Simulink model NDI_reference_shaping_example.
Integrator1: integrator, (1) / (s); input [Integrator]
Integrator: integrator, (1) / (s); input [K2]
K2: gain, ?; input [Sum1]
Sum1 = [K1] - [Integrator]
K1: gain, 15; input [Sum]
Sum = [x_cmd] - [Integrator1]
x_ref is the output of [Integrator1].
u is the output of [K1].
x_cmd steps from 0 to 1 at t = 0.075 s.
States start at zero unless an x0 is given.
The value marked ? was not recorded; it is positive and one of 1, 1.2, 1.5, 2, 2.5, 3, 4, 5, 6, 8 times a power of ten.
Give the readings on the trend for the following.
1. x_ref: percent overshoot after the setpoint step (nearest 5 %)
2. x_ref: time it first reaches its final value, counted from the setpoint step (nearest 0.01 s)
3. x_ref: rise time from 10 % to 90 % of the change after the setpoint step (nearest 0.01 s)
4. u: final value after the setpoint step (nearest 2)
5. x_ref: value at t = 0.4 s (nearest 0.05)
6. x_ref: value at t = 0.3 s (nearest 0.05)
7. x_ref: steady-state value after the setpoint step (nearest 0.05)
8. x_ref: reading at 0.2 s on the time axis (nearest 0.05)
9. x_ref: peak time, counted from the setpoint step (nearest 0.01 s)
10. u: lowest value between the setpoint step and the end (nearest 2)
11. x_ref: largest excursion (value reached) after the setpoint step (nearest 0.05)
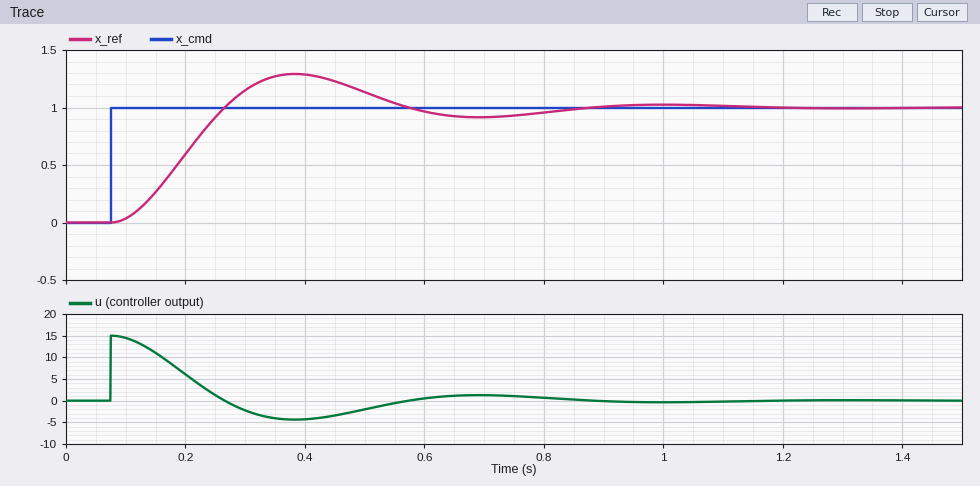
30 %
0.19 s
0.13 s
0
1.30
1.15
1.00
0.60
0.31 s
-4
1.30
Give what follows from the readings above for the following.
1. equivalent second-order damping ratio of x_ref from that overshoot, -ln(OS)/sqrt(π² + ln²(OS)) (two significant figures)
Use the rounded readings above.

0.36
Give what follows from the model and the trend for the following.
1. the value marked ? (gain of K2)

8
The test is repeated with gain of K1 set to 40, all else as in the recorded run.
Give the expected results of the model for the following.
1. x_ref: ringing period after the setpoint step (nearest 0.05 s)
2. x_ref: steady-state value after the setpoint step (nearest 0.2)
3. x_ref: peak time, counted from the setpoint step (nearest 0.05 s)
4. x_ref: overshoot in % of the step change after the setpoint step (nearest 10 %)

0.35 s
1.0
0.20 s
50 %
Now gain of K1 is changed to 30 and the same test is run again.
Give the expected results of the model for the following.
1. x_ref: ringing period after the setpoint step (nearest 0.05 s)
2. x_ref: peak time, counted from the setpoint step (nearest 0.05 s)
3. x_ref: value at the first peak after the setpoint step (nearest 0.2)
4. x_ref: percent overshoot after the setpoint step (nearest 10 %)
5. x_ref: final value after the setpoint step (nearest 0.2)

0.40 s
0.20 s
1.4
40 %
1.0
